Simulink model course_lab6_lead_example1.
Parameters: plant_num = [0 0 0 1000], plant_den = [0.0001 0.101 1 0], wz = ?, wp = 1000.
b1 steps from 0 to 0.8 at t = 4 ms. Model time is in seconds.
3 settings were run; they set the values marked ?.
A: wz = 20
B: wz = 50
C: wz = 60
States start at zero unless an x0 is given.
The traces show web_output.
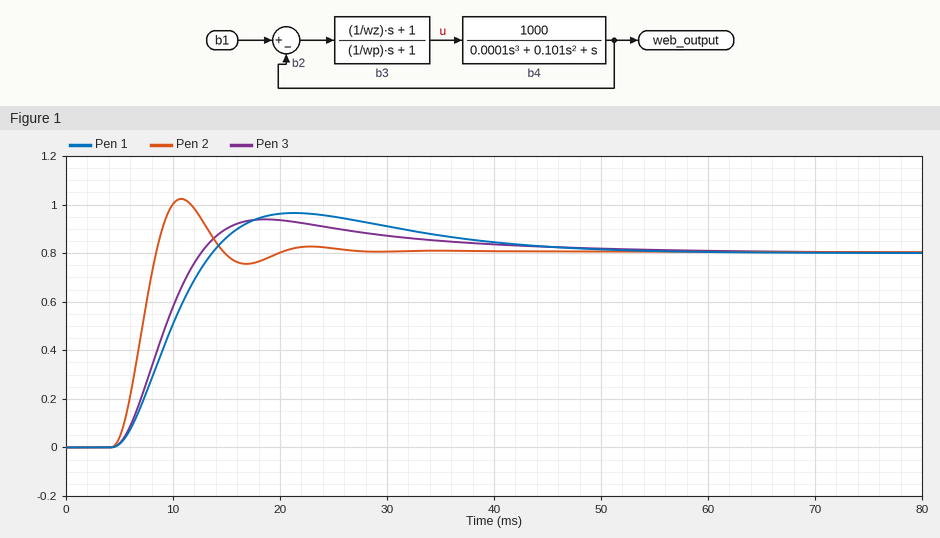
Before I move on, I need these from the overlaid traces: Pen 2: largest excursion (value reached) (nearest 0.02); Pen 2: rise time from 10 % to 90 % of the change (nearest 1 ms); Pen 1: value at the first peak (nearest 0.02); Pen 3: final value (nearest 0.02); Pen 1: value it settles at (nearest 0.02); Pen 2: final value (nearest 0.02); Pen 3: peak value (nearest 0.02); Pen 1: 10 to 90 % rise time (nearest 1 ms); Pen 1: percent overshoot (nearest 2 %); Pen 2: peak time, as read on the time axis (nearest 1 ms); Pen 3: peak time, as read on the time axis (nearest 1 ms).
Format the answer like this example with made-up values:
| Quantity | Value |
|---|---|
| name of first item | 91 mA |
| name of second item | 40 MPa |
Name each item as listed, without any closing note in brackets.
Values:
| Quantity | Value |
|---|---|
| Pen 2: largest excursion (value reached) | 1.02 |
| Pen 2: rise time from 10 % to 90 % of the change | 3 ms |
| Pen 1: value at the first peak | 0.96 |
| Pen 3: final value | 0.80 |
| Pen 1: value it settles at | 0.80 |
| Pen 2: final value | 0.80 |
| Pen 3: peak value | 0.94 |
| Pen 1: 10 to 90 % rise time | 6 ms |
| Pen 1: percent overshoot | 20 % |
| Pen 2: peak time, as read on the time axis | 11 ms |
| Pen 3: peak time, as read on the time axis | 19 ms |
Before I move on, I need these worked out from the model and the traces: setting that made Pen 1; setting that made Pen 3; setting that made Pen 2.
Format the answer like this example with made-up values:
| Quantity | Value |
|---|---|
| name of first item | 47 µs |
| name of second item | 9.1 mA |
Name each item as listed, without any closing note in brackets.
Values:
| Quantity | Value |
|---|---|
| setting that made Pen 1 | C |
| setting that made Pen 3 | B |
| setting that made Pen 2 | A |
